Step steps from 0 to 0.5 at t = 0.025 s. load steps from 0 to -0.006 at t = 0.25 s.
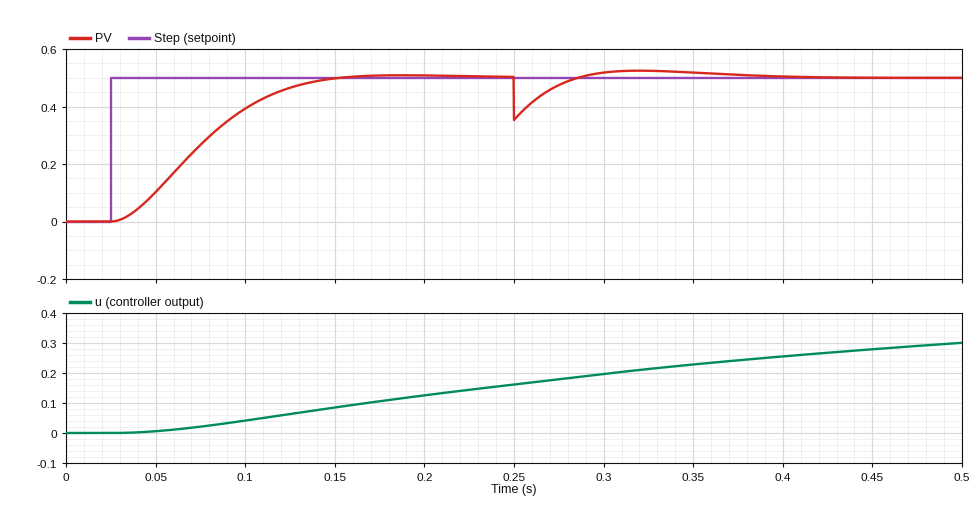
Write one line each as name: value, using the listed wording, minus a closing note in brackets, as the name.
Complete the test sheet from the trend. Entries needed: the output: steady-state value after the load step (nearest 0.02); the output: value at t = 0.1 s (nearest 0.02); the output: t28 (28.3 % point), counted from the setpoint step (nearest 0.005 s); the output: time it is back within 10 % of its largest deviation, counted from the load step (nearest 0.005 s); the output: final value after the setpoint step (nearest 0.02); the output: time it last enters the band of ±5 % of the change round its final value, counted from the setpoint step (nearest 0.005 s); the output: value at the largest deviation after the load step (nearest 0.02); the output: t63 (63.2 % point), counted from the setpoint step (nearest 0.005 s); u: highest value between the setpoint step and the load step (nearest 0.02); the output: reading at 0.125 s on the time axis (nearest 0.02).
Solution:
the output: steady-state value after the load step: 0.50
the output: value at t = 0.1 s: 0.40
the output: t28 (28.3 % point), counted from the setpoint step: 0.030 s
the output: time it is back within 10 % of its largest deviation, counted from the load step: 0.110 s
the output: final value after the setpoint step: 0.50
the output: time it last enters the band of ±5 % of the change round its final value, counted from the setpoint step: 0.105 s
the output: value at the largest deviation after the load step: 0.36
the output: t63 (63.2 % point), counted from the setpoint step: 0.060 s
u: highest value between the setpoint step and the load step: 0.16
the output: reading at 0.125 s on the time axis: 0.46
